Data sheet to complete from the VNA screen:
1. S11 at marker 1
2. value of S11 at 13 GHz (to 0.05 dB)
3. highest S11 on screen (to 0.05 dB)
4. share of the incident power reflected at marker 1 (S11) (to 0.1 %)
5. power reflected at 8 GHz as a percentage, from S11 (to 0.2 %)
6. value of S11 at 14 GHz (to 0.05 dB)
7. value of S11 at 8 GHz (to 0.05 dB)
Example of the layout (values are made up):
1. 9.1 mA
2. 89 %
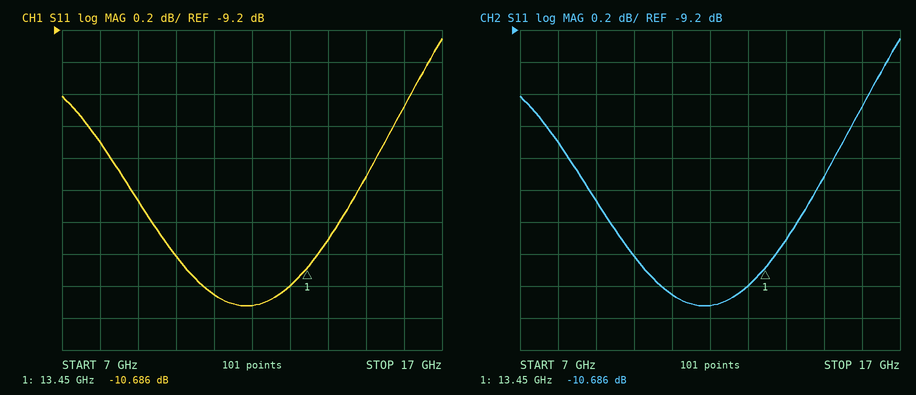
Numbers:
1. -10.686 dB
2. -10.80 dB
3. -9.25 dB
4. 8.5 %
5. 10.2 %
6. -10.50 dB
7. -9.90 dB
